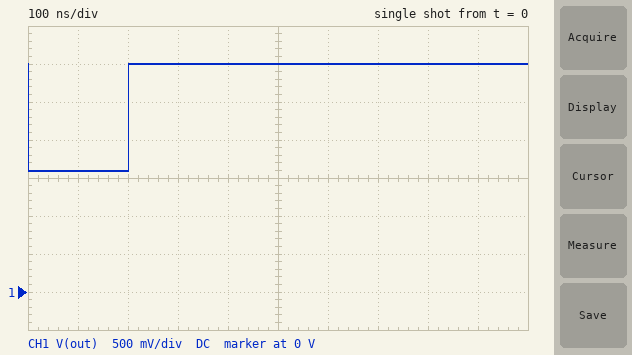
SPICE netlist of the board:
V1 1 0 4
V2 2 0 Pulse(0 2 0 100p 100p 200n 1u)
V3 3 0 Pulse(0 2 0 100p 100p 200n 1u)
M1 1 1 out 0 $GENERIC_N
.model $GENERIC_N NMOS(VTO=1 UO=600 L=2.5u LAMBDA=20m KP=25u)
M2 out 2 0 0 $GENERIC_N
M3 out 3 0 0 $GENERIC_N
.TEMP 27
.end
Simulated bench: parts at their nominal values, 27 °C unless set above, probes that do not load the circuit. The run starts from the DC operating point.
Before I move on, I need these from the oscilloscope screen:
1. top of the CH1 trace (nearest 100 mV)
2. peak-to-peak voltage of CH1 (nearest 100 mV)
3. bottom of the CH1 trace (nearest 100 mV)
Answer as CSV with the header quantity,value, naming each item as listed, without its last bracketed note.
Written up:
quantity,value
top of the CH1 trace,3.0 V
peak-to-peak voltage of CH1,1.4 V
bottom of the CH1 trace,1.6 V
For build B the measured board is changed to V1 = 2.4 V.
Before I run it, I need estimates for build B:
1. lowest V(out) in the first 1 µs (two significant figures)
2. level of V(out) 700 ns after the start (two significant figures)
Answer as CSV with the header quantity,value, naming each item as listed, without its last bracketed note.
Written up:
quantity,value
lowest V(out) in the first 1 µs,350 mV
level of V(out) 700 ns after the start,1.4 V
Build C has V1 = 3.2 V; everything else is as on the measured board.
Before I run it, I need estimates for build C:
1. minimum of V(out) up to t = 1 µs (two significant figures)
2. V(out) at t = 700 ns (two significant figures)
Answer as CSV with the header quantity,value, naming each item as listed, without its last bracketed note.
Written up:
quantity,value
minimum of V(out) up to t = 1 µs,830 mV
V(out) at t = 700 ns,2.2 V
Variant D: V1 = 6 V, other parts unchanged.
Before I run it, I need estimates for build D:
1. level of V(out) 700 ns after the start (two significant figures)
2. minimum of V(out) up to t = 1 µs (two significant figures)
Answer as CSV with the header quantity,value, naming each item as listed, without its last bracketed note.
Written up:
quantity,value
level of V(out) 700 ns after the start,5.0 V
minimum of V(out) up to t = 1 µs,3.6 V
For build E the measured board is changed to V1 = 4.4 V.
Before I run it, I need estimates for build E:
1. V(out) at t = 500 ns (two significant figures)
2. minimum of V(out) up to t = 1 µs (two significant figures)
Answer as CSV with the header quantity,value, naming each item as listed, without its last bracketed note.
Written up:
quantity,value
V(out) at t = 500 ns,3.4 V
minimum of V(out) up to t = 1 µs,2.0 V
